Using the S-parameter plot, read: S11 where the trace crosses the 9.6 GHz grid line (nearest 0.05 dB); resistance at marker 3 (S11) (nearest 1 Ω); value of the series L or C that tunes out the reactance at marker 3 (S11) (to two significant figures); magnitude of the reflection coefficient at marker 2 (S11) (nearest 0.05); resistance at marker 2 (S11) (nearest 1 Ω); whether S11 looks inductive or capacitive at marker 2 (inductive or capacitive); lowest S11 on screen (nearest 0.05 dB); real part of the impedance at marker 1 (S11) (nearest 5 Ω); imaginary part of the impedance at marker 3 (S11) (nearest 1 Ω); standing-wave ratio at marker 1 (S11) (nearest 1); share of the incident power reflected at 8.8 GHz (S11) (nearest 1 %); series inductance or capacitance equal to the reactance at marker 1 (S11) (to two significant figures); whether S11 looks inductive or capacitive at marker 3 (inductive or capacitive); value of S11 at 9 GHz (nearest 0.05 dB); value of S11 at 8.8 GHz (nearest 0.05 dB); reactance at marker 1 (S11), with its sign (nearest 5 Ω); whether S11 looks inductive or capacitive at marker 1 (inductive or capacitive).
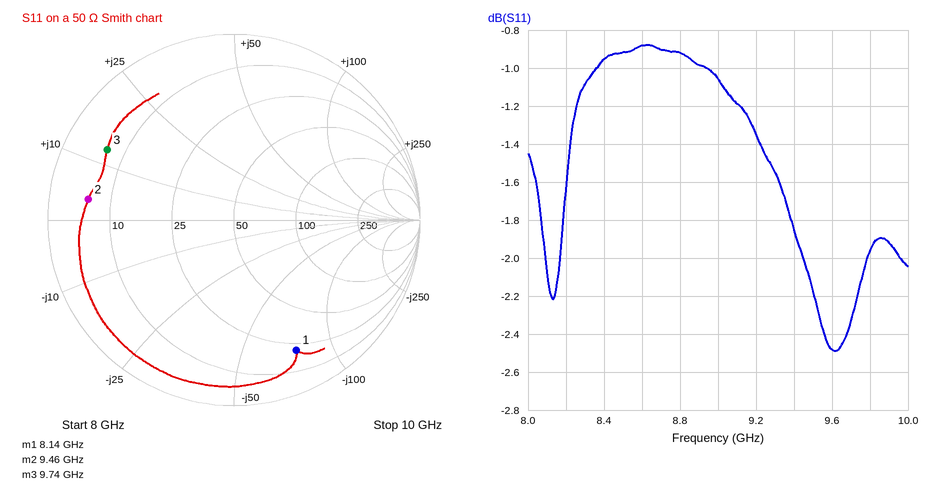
-2.50 dB
7 Ω
1.3 pF
0.80
6 Ω
inductive
-2.50 dB
20 Ω
+13 Ω
8
81 %
260 fF
inductive
-1.05 dB
-0.90 dB
-75 Ω
capacitive
